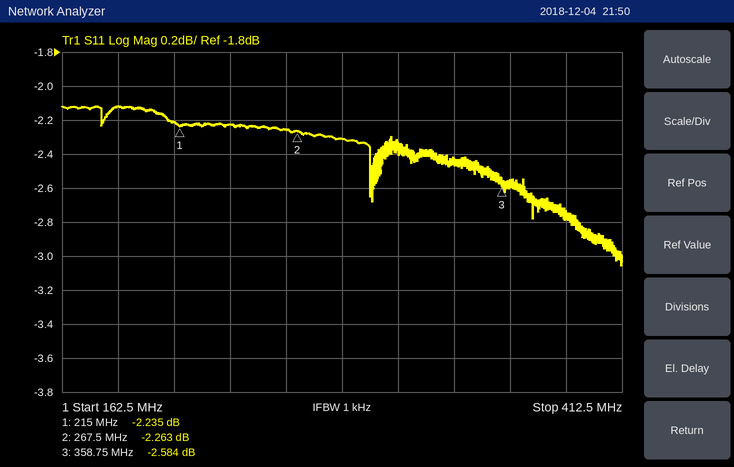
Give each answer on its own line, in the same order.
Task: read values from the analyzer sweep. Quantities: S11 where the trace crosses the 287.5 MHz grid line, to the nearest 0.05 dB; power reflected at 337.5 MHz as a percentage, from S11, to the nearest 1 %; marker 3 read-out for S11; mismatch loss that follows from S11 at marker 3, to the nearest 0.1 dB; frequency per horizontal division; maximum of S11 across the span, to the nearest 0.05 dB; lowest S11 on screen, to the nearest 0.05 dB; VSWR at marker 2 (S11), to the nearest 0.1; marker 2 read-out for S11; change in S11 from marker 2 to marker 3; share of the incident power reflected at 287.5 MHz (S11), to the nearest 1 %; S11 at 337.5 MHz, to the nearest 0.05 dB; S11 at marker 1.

-2.30 dB
57 %
-2.584 dB
3.5 dB
25 MHz
-2.10 dB
-3.05 dB
7.7
-2.263 dB
-0.321 dB
59 %
-2.45 dB
-2.235 dB
